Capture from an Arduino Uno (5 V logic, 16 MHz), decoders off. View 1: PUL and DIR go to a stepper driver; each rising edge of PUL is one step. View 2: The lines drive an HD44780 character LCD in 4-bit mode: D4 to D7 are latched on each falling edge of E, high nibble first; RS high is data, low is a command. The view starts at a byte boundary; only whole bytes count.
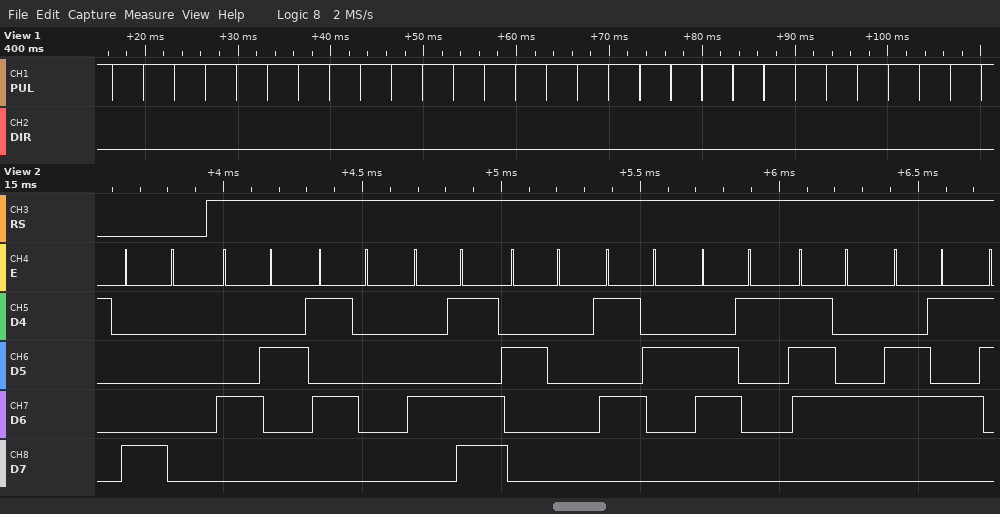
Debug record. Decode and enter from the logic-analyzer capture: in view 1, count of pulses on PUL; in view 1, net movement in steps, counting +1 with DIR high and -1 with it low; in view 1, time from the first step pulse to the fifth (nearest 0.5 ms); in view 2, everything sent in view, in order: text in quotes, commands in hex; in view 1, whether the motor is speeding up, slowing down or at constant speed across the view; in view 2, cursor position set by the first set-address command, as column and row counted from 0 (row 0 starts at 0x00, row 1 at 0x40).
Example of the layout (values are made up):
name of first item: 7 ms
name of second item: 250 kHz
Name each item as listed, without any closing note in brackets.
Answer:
in view 1, count of pulses on PUL: 29
in view 1, net movement in steps, counting +1 with DIR high and -1 with it low: -29
in view 1, time from the first step pulse to the fifth: 13.5 ms
in view 2, everything sent in view, in order: text in quotes, commands in hex: 0x80 "BPM Rate"
in view 1, whether the motor is speeding up, slowing down or at constant speed across the view: constant speed
in view 2, cursor position set by the first set-address command, as column and row counted from 0: column 0, row 0
